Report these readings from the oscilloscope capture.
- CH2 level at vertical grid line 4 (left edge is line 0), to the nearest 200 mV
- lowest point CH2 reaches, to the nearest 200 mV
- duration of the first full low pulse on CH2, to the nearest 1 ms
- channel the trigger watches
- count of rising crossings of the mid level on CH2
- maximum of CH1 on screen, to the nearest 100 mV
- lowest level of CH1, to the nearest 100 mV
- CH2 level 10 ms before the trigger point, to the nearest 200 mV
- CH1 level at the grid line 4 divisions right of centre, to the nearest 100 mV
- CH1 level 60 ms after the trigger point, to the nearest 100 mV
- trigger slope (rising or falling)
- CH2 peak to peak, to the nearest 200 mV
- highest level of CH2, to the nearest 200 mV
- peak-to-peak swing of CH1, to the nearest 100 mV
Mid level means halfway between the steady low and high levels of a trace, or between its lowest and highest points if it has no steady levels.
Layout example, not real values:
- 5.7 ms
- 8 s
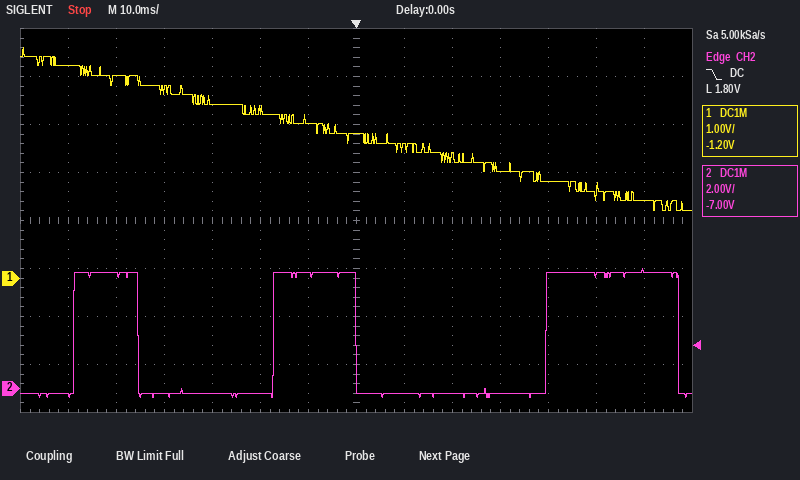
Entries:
- -200 mV
- -400 mV
- 28 ms
- CH2
- 3
- 4.8 V
- 1.4 V
- 4.8 V
- 2.0 V
- 1.6 V
- falling
- 5.4 V
- 5.0 V
- 3.4 V
